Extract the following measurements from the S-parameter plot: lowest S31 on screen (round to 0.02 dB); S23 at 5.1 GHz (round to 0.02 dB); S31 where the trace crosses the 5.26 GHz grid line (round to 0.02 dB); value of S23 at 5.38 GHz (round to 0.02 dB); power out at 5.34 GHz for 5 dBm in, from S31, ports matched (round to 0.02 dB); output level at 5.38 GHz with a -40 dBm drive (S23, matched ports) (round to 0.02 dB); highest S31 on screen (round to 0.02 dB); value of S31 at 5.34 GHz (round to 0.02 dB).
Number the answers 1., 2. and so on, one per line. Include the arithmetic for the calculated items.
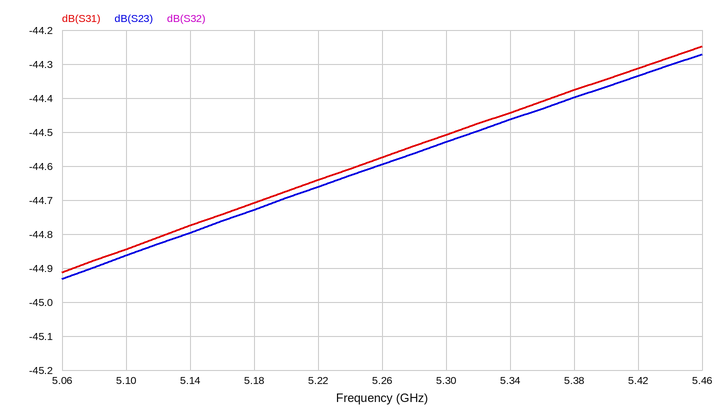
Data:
1. -44.92 dB
2. -44.86 dB
3. -44.58 dB
4. -44.40 dB
5. 5 dBm + (-44.44 dB) = -39.44 dBm
6. -40 dBm + (-44.40 dB) = -84.40 dBm
7. -44.24 dB
8. -44.44 dB
